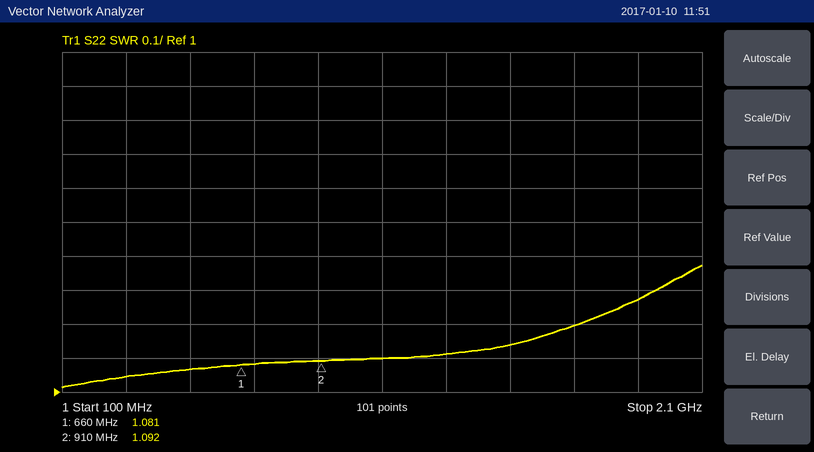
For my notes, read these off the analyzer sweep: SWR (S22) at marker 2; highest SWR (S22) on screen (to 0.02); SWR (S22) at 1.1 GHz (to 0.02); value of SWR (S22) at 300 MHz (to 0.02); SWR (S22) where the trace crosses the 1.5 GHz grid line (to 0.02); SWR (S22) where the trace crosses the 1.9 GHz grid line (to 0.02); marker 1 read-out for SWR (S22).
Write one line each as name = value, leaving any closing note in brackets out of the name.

SWR (S22) at marker 2 = 1.092
highest SWR (S22) on screen = 1.38
SWR (S22) at 1.1 GHz = 1.10
value of SWR (S22) at 300 MHz = 1.04
SWR (S22) where the trace crosses the 1.5 GHz grid line = 1.14
SWR (S22) where the trace crosses the 1.9 GHz grid line = 1.28
marker 1 read-out for SWR = 1.081
